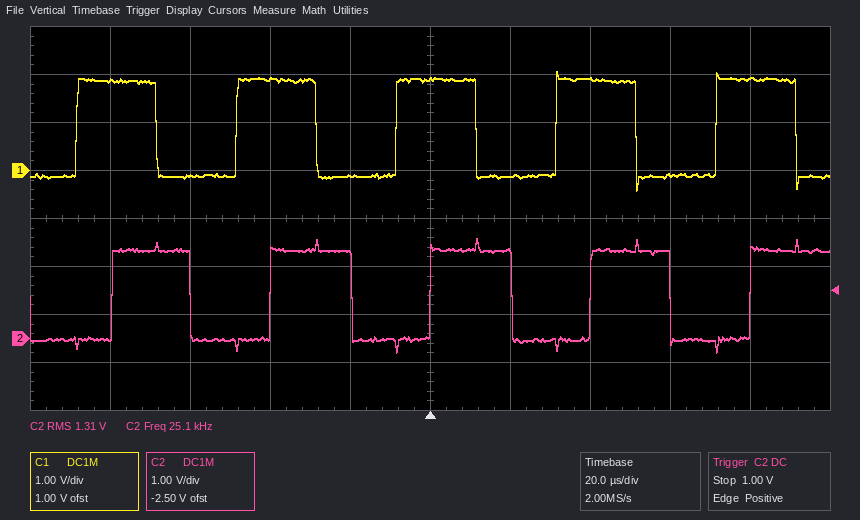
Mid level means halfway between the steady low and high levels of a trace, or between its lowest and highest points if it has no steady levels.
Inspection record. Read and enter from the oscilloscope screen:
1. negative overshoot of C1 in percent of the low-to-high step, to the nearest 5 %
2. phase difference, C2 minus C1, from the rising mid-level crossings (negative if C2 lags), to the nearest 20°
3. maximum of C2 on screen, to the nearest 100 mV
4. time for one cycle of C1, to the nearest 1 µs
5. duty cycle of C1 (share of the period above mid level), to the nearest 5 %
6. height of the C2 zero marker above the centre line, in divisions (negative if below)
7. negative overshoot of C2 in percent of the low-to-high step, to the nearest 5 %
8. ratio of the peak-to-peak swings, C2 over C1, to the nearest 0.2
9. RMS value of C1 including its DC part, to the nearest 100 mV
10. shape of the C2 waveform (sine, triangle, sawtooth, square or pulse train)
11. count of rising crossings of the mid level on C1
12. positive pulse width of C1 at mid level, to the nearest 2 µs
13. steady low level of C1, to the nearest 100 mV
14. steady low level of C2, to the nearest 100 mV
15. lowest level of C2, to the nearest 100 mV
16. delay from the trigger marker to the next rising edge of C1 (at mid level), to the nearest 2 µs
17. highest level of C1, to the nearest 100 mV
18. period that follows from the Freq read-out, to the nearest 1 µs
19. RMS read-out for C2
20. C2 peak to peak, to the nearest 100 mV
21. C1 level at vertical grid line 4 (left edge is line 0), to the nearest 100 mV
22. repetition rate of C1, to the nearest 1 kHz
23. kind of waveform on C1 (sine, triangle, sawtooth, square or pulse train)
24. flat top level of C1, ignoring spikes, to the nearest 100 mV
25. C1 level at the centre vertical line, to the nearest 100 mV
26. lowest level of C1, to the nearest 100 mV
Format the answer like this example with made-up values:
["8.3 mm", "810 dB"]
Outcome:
["15 %", "-80°", "2.1 V", "40 µs", "50 %", "-2.5 div", "15 %", "1.0", "1.3 V", "square", "5", "20 µs", "-100 mV", "0.0 V", "-300 mV", "32 µs", "2.1 V", "40 µs", "1.31 V", "2.4 V", "-100 mV", "25 kHz", "square", "1.9 V", "1.9 V", "-400 mV"]
